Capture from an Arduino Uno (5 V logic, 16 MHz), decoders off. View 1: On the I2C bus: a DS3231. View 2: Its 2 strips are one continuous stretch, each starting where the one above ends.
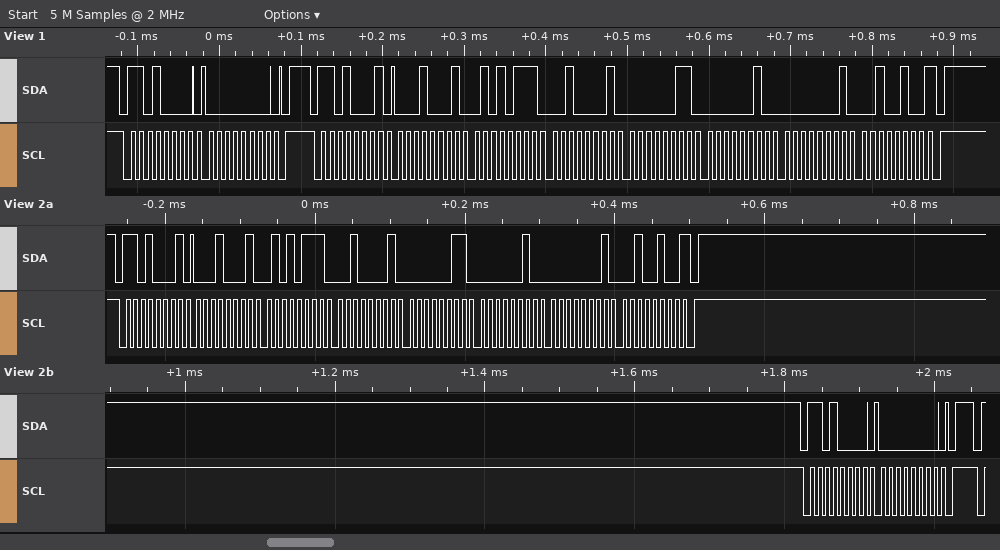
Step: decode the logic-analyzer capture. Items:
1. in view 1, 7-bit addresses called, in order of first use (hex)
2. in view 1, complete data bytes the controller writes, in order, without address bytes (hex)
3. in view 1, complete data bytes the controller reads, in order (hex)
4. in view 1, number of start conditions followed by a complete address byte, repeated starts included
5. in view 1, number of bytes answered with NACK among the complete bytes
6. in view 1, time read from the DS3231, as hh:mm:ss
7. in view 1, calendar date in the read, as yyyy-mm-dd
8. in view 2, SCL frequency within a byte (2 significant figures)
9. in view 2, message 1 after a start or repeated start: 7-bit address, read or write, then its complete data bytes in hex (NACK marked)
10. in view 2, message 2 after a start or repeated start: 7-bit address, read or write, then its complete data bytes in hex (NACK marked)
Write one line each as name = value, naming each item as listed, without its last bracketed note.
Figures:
in view 1, 7-bit addresses called, in order of first use = 0x68
in view 1, complete data bytes the controller writes, in order, without address bytes = 00
in view 1, complete data bytes the controller reads, in order = 11 57 21 03 02 01 24
in view 1, number of start conditions followed by a complete address byte, repeated starts included = 2
in view 1, number of bytes answered with NACK among the complete bytes = 1
in view 1, time read from the DS3231, as hh:mm:ss = 21:57:11
in view 1, calendar date in the read, as yyyy-mm-dd = 2024-01-02
in view 2, SCL frequency within a byte = 100 kHz
in view 2, message 1 after a start or repeated start: 7-bit address, read or write, then its complete data bytes in hex = 0x68 read: 11 57 21 03 02 01 24 NACK
in view 2, message 2 after a start or repeated start: 7-bit address, read or write, then its complete data bytes in hex = 0x68 write: 00
